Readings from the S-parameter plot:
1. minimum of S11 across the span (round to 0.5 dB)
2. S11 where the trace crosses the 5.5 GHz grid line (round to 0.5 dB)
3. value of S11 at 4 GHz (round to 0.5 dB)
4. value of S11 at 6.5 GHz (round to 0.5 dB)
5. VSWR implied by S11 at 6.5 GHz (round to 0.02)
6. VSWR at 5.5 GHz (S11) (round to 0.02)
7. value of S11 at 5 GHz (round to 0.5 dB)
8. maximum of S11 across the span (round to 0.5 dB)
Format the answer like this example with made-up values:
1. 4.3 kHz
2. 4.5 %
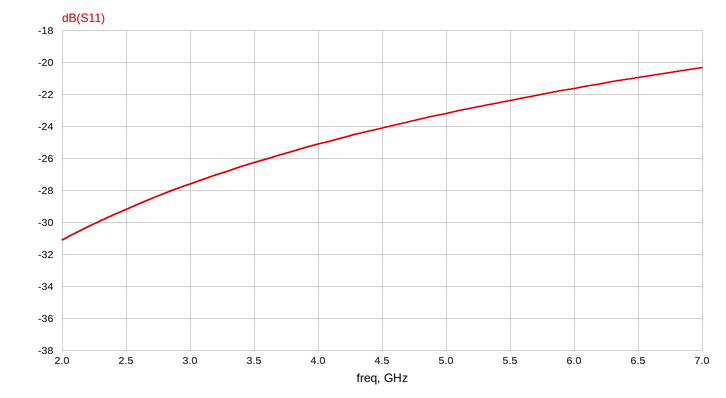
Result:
1. -31.0 dB
2. -22.5 dB
3. -25.0 dB
4. -21.0 dB
5. 1.20
6. 1.16
7. -23.0 dB
8. -20.5 dB
